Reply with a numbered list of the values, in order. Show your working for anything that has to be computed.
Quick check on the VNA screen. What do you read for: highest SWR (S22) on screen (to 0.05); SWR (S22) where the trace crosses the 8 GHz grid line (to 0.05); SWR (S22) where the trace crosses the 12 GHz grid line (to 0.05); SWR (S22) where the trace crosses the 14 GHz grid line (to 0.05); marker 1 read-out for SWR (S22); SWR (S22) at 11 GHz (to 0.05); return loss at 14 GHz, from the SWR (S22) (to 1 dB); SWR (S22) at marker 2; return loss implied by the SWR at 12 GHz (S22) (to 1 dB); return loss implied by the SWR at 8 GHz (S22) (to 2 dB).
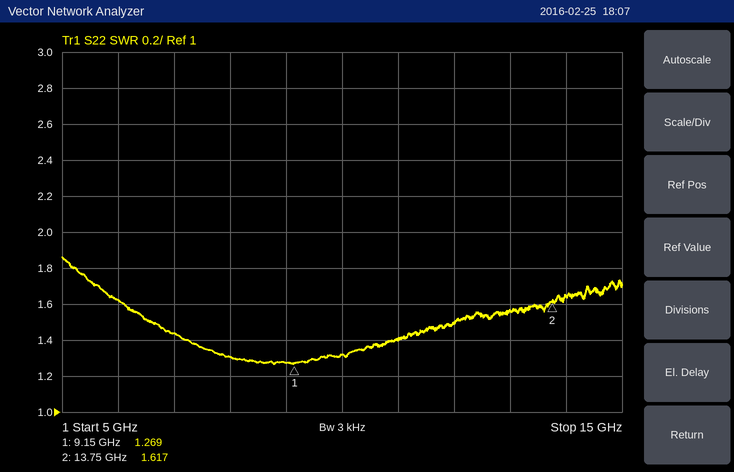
1. 1.85
2. 1.30
3. 1.50
4. 1.65
5. 1.269
6. 1.40
7. −20 log10((1.65 − 1)/(1.65 + 1)) ≈ 12 dB
8. 1.617
9. −20 log10((1.5 − 1)/(1.5 + 1)) ≈ 14 dB
10. −20 log10((1.3 − 1)/(1.3 + 1)) ≈ 18 dB
